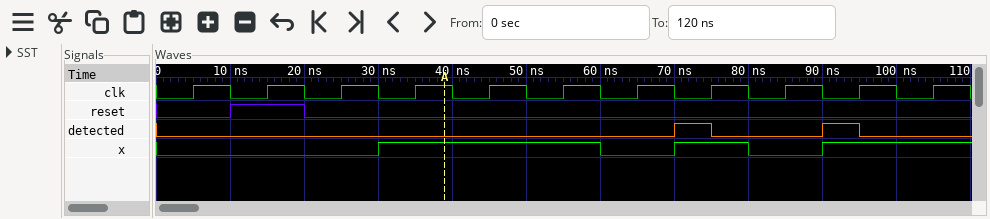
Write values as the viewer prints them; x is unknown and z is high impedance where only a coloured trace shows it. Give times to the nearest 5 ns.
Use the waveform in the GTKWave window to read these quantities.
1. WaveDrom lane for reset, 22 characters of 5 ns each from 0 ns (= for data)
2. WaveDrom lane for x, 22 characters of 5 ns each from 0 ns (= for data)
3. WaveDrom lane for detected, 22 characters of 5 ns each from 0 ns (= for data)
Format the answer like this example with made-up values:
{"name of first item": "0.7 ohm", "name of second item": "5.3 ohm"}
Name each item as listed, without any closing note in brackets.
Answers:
{"WaveDrom lane for reset, 22 characters of 5 ns each from 0 ns": "{name: 'reset', wave: '0.1.0.................'}", "WaveDrom lane for x, 22 characters of 5 ns each from 0 ns": "{name: 'x', wave: '0.....1.....0.1.0.1...'}", "WaveDrom lane for detected, 22 characters of 5 ns each from 0 ns": "{name: 'detected', wave: '0.............10..10..'}"}
